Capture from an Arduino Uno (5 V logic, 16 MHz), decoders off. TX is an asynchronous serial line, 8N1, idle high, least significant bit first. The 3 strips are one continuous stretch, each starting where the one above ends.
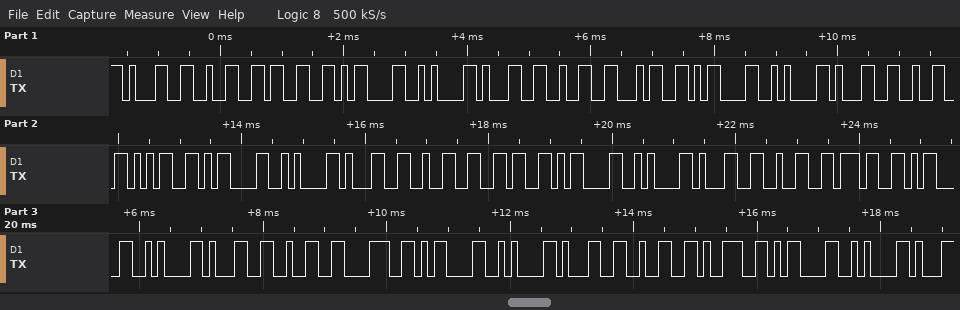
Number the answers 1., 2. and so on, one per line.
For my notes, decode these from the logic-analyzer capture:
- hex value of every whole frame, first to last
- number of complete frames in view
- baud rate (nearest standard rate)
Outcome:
1. 0x31 0x32 0x33 0x0D 0x0A 0x31 0x32 0x34 0x0D 0x0A 0x31 0x32 0x35 0x0D 0x0A 0x31 0x32 0x36 0x0D 0x0A 0x31 0x32 0x37 0x0D 0x0A 0x31 0x32 0x38 0x0D 0x0A 0x31 0x32 0x39 0x0D 0x0A
2. 35
3. 9600 baud
